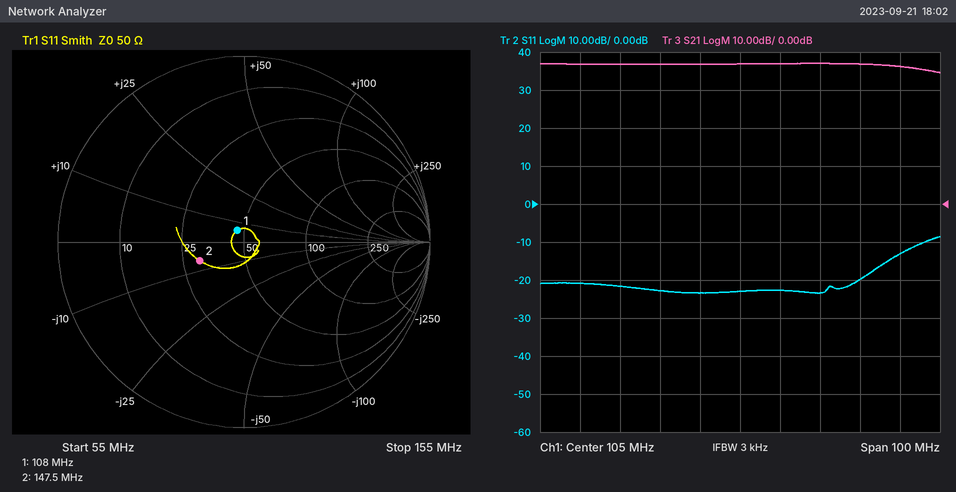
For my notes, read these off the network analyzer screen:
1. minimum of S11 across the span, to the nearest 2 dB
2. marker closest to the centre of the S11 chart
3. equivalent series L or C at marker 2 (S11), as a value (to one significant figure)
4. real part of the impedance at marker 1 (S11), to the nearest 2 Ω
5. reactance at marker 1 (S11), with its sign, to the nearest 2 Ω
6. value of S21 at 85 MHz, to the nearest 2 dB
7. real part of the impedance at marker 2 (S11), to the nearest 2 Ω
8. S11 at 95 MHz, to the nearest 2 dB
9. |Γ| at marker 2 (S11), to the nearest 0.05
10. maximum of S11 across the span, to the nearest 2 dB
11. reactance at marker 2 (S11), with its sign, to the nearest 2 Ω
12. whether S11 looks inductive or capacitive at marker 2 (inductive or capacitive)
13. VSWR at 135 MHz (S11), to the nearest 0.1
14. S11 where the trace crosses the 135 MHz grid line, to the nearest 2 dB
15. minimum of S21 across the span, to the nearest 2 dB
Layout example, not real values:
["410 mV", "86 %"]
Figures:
["-24 dB", "marker 1", "200 pF", "46 Ω", "+6 Ω", "36 dB", "30 Ω", "-24 dB", "0.25", "-8 dB", "-6 Ω", "capacitive", "1.2", "-20 dB", "34 dB"]
